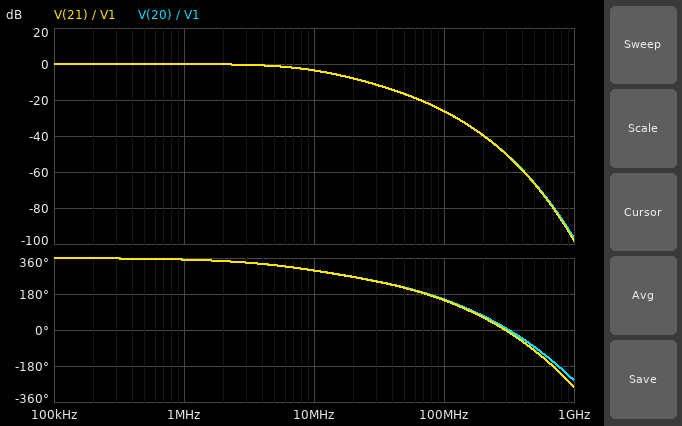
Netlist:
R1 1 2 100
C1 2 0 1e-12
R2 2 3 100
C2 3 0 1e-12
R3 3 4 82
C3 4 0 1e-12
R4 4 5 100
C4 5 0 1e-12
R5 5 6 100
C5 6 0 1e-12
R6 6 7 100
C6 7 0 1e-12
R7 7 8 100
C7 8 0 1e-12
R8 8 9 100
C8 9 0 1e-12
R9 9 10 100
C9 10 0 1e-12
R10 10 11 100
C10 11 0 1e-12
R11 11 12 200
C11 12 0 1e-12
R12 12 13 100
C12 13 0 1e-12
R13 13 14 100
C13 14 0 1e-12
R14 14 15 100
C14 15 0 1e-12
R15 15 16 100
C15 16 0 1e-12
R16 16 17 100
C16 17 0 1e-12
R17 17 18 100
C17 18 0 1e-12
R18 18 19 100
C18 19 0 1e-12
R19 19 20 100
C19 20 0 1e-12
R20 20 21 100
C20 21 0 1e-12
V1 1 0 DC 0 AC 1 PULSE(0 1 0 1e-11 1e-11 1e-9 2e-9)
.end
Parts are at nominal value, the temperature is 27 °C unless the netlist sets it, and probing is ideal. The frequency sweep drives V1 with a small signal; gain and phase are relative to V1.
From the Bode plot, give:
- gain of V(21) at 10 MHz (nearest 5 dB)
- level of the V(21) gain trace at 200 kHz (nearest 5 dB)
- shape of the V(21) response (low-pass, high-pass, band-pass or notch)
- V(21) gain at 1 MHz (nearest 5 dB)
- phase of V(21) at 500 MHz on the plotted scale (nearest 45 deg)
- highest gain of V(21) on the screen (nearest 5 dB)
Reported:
-5 dB
0 dB
low-pass
0 dB
-90 deg
0 dB
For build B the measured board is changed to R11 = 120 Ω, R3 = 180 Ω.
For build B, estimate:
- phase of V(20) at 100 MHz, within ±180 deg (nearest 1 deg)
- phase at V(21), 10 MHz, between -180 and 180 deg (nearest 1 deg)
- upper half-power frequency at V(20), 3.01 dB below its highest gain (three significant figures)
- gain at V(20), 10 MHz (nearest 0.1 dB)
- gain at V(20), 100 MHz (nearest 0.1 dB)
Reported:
152 deg
-64 deg
8.49 MHz
-3.8 dB
-26.7 dB
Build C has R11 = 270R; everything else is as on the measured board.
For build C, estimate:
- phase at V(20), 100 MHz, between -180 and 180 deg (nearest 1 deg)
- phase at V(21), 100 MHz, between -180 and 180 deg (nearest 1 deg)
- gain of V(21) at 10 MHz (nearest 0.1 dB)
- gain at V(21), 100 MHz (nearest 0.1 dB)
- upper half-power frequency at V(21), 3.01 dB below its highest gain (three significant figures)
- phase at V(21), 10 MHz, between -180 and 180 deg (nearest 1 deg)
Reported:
150 deg
146 deg
-3.7 dB
-26.7 dB
8.64 MHz
-64 deg
